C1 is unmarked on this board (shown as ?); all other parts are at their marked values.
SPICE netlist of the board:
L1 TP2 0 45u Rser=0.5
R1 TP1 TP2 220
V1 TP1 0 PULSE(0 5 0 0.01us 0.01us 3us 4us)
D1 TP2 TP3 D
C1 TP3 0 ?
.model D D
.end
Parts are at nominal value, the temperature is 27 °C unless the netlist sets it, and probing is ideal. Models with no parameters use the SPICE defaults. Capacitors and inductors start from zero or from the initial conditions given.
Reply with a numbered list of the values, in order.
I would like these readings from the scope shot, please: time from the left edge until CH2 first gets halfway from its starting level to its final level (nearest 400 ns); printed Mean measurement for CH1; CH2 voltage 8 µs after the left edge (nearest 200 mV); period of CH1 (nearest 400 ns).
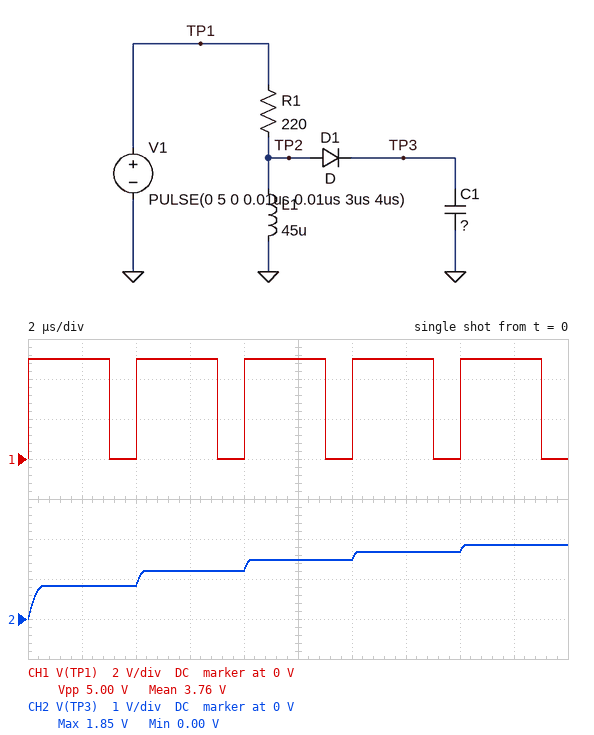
1. 4.0 µs
2. 3.76 V
3. 1.2 V
4. 4.0 µs
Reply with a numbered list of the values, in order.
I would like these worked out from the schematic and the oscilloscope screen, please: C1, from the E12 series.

1. 6.8 nF
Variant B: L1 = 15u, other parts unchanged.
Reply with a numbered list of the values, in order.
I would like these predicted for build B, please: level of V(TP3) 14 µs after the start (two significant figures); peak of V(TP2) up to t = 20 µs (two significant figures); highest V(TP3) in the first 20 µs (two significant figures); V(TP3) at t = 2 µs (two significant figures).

1. 980 mV
2. 1.8 V
3. 1.1 V
4. 390 mV
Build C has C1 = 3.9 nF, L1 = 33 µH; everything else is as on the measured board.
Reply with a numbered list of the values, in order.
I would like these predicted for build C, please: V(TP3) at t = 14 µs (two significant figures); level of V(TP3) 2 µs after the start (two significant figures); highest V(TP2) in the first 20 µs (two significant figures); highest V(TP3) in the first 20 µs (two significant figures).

1. 1.9 V
2. 940 mV
3. 2.7 V
4. 2.0 V
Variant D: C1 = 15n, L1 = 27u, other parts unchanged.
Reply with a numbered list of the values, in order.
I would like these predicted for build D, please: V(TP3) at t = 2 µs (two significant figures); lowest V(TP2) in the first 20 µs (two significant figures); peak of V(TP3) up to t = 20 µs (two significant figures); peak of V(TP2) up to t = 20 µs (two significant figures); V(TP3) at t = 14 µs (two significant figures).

1. 340 mV
2. -4.8 V
3. 1.0 V
4. 1.7 V
5. 880 mV
